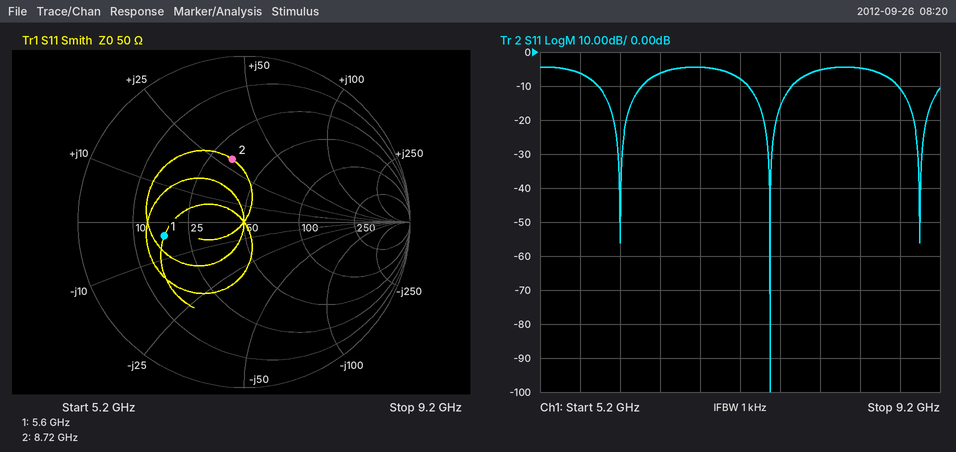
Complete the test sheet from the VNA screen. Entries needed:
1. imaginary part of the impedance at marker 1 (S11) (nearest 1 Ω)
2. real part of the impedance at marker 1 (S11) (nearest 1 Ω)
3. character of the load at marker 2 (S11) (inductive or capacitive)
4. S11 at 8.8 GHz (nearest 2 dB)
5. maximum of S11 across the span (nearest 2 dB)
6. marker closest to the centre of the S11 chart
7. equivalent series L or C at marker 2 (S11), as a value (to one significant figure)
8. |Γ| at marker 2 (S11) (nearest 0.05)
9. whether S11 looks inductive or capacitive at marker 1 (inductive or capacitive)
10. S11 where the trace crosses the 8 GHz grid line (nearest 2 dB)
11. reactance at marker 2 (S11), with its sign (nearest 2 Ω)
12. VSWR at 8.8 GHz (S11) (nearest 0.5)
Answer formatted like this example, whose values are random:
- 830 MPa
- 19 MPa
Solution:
- -4 Ω
- 17 Ω
- inductive
- -10 dB
- -4 dB
- marker 2
- 500 pH
- 0.40
- capacitive
- -6 dB
- +30 Ω
- 2.0
